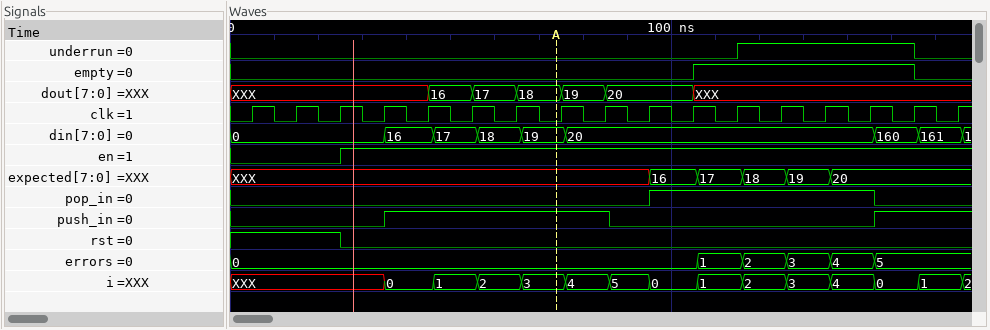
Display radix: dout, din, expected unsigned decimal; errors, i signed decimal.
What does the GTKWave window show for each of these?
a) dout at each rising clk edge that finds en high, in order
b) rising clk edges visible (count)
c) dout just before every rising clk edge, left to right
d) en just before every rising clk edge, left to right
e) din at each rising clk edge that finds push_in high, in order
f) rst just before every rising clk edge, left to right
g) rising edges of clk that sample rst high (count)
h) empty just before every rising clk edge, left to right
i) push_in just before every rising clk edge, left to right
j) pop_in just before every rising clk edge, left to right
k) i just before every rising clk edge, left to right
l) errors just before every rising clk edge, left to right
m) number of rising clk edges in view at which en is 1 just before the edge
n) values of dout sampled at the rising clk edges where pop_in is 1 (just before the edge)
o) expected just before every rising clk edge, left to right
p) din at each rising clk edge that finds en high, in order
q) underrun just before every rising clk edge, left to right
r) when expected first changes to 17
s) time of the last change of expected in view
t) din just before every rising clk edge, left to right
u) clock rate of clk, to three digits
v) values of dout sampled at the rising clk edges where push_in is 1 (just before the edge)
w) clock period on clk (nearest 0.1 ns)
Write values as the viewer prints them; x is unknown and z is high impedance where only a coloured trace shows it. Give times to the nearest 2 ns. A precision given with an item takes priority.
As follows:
XXX, XXX, 16, 17, 18, 19, 20, 20, XXX, XXX, XXX, XXX, XXX, XXX
17
XXX, XXX, XXX, XXX, XXX, 16, 17, 18, 19, 20, 20, XXX, XXX, XXX, XXX, XXX, XXX
0 0 0 1 1 1 1 1 1 1 1 1 1 1 1 1 1
16, 17, 18, 19, 20, 160, 161
1 1 1 0 0 0 0 0 0 0 0 0 0 0 0 0 0
3
0 0 0 0 0 0 0 0 0 0 0 1 1 1 1 1 0
0 0 0 0 1 1 1 1 1 0 0 0 0 0 0 1 1
0 0 0 0 0 0 0 0 0 0 1 1 1 1 1 0 0
XXX, XXX, XXX, XXX, 0, 1, 2, 3, 4, 5, 0, 1, 2, 3, 4, 0, 1
0, 0, 0, 0, 0, 0, 0, 0, 0, 0, 0, 1, 2, 3, 4, 5, 5
14
20, XXX, XXX, XXX, XXX
XXX, XXX, XXX, XXX, XXX, XXX, XXX, XXX, XXX, XXX, 16, 17, 18, 19, 20, 20, 20
0, 16, 17, 18, 19, 20, 20, 20, 20, 20, 20, 20, 160, 161
0 0 0 0 0 0 0 0 0 0 0 0 1 1 1 1 0
106 ns
136 ns
0, 0, 0, 0, 16, 17, 18, 19, 20, 20, 20, 20, 20, 20, 20, 160, 161
100 MHz
XXX, 16, 17, 18, 19, XXX, XXX
10 ns
